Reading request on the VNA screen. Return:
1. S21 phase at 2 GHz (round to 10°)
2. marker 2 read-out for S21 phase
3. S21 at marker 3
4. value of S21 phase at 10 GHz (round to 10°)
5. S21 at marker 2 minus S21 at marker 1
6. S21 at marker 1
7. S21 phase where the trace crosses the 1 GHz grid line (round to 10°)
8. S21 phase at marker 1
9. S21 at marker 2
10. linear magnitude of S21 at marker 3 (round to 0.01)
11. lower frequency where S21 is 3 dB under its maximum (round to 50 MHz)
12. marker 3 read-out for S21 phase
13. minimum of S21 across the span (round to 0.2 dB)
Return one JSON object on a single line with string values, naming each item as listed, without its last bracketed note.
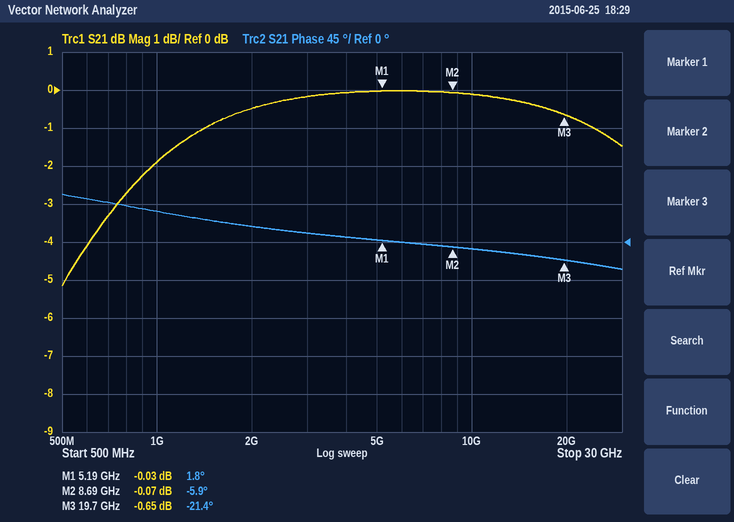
{"S21 phase at 2 GHz": "20°", "marker 2 read-out for S21 phase": "-5.9°", "S21 at marker 3": "-0.65 dB", "value of S21 phase at 10 GHz": "-10°", "S21 at marker 2 minus S21 at marker 1": "-0.04 dB", "S21 at marker 1": "-0.03 dB", "S21 phase where the trace crosses the 1 GHz grid line": "40°", "S21 phase at marker 1": "1.8°", "S21 at marker 2": "-0.07 dB", "linear magnitude of S21 at marker 3": "0.93", "lower frequency where S21 is 3 dB under its maximum": "750 MHz", "marker 3 read-out for S21 phase": "-21.4°", "minimum of S21 across the span": "-5.2 dB"}
